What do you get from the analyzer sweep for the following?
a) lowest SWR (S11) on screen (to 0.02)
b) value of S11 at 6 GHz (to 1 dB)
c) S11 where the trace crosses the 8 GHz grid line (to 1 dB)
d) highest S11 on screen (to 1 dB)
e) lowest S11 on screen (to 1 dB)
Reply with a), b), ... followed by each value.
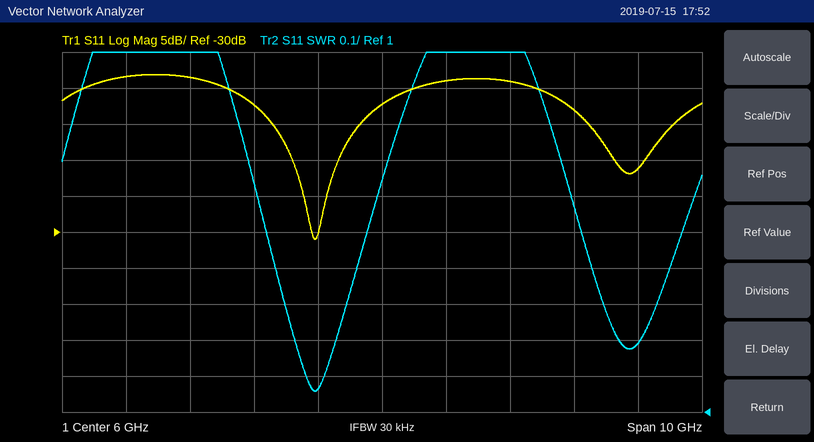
a) 1.06
b) -12 dB
c) -9 dB
d) -8 dB
e) -31 dB
